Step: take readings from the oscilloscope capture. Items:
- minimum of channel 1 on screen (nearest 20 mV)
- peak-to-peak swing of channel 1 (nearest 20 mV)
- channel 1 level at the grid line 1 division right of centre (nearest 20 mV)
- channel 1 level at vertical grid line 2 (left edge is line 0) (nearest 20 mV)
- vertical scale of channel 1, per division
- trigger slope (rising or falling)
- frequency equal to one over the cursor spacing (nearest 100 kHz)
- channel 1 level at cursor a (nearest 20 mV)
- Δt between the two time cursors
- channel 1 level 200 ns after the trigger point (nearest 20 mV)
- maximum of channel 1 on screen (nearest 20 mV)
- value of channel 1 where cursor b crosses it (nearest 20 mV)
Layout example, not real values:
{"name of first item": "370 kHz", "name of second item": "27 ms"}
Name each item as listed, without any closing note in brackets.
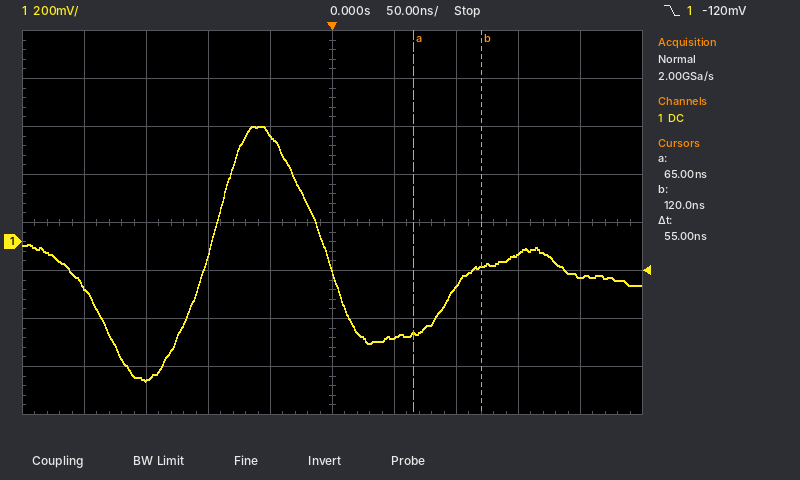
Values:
{"minimum of channel 1 on screen": "-580 mV", "peak-to-peak swing of channel 1": "1.06 V", "channel 1 level at the grid line 1 division right of centre": "-400 mV", "channel 1 level at vertical grid line 2 (left edge is line 0)": "-580 mV", "vertical scale of channel 1, per division": "200 mV", "trigger slope": "falling", "frequency equal to one over the cursor spacing": "18.2 MHz", "channel 1 level at cursor a": "-380 mV", "Δt between the two time cursors": "55 ns", "channel 1 level 200 ns after the trigger point": "-140 mV", "maximum of channel 1 on screen": "480 mV", "value of channel 1 where cursor b crosses it": "-100 mV"}
